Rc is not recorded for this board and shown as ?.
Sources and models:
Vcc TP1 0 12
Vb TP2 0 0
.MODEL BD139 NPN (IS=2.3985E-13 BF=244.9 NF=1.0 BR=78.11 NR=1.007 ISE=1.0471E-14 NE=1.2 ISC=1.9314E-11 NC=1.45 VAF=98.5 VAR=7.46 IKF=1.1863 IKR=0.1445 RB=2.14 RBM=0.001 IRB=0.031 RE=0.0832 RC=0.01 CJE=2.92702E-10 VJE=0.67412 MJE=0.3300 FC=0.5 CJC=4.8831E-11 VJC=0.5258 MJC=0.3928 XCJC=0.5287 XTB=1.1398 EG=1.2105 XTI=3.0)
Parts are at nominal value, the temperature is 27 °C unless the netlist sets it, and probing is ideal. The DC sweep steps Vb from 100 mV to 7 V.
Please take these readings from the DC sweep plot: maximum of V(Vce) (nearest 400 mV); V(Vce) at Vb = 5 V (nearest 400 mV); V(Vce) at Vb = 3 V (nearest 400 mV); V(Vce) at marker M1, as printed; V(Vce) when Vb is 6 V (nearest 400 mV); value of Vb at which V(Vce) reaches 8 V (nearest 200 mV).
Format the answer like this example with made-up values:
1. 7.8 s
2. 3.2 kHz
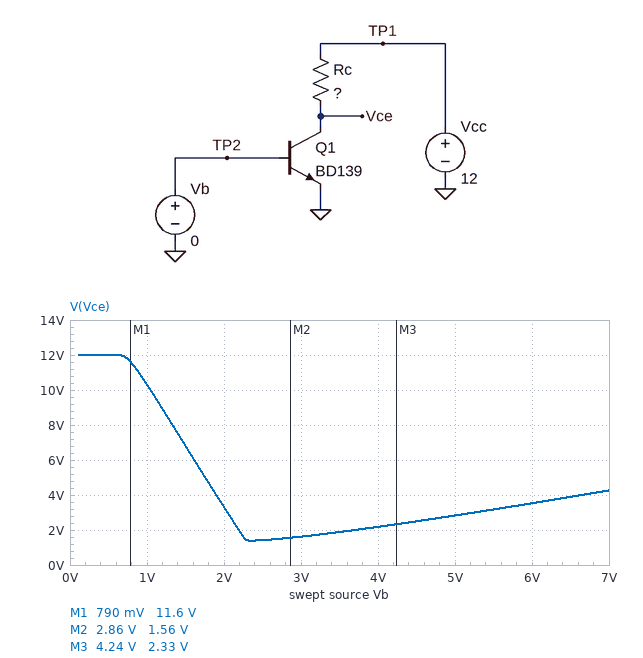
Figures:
1. 12.0 V
2. 2.8 V
3. 1.6 V
4. 11.6 V
5. 3.6 V
6. 1.4 V
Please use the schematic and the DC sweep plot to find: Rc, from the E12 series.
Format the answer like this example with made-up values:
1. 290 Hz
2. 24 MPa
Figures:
1. 0.82 Ω
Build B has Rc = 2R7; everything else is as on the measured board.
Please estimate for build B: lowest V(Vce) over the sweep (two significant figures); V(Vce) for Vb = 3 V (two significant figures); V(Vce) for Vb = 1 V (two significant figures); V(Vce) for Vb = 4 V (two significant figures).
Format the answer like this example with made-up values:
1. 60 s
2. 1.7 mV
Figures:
1. 480 mV
2. 1.2 V
3. 6.5 V
4. 1.9 V
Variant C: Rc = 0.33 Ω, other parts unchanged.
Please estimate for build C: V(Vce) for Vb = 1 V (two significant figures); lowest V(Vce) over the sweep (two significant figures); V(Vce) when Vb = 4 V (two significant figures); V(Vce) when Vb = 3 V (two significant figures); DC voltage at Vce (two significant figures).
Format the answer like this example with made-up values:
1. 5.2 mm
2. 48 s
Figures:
1. 11 V
2. 3.0 V
3. 3.1 V
4. 5.7 V
5. 12 V
